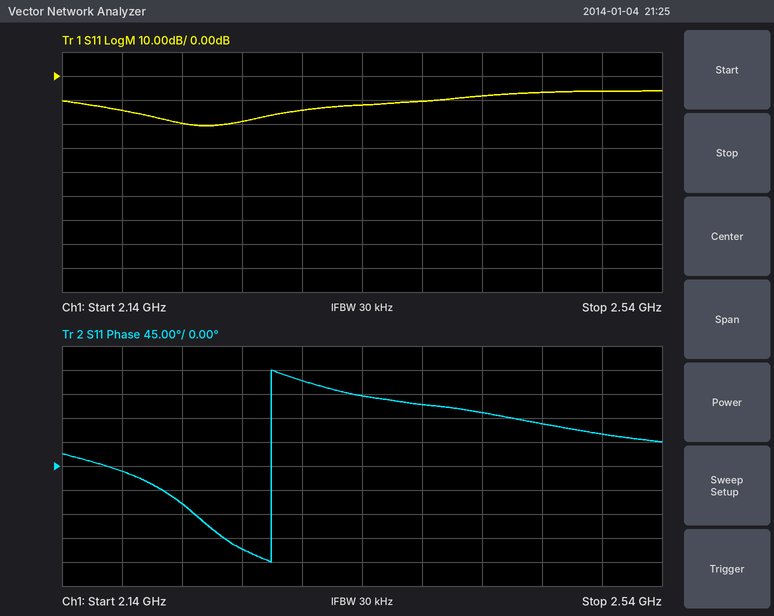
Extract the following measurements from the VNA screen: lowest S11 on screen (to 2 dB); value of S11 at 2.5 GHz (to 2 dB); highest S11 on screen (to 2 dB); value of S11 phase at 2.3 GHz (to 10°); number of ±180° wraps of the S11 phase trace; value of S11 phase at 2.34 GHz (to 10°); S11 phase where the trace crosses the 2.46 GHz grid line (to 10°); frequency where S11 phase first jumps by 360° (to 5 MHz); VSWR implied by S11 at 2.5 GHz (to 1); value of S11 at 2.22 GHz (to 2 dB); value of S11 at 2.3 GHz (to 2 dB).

-20 dB
-6 dB
-6 dB
160°
1
130°
80°
2.280 GHz
3
-20 dB
-14 dB
